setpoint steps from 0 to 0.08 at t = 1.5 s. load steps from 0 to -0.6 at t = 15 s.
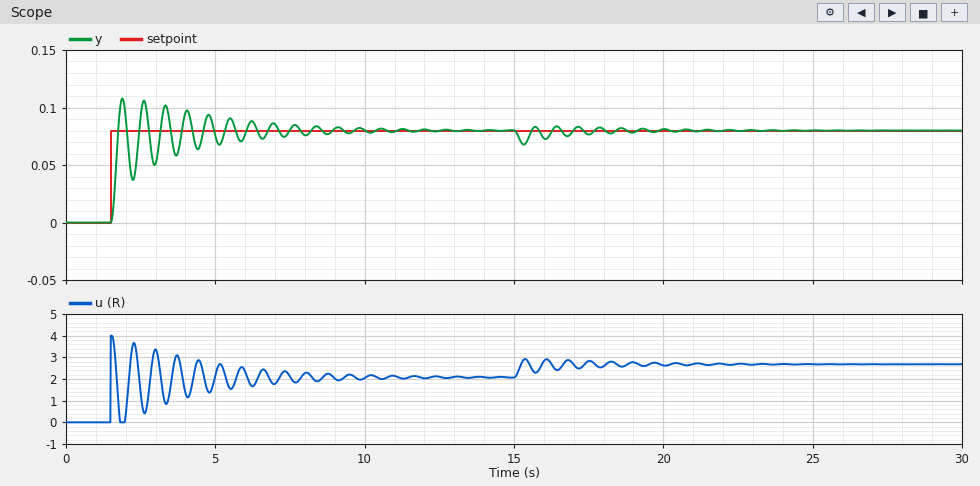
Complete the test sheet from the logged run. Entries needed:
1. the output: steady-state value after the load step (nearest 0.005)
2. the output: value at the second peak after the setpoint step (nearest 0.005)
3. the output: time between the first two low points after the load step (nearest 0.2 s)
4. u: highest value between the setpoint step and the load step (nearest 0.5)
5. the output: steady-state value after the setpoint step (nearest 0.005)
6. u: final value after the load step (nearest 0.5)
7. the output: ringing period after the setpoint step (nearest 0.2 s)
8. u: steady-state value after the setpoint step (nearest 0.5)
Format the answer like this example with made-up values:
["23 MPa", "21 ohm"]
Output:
["0.080", "0.105", "0.8 s", "4.0", "0.080", "2.5", "0.8 s", "2.0"]
